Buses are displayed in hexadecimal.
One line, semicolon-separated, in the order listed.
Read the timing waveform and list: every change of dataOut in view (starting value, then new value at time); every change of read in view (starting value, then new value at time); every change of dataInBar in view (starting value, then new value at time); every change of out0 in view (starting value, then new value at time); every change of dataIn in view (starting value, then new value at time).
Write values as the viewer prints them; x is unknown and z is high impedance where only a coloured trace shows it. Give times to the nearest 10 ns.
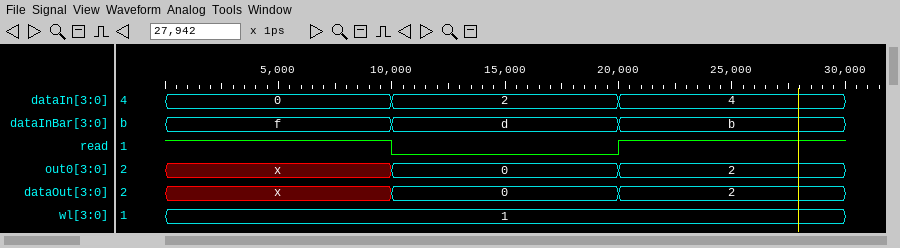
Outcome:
x, 0 at 10 ns, 2 at 20 ns; 1, 0 at 10 ns, 1 at 20 ns; f, d at 10 ns, b at 20 ns; x, 0 at 10 ns, 2 at 20 ns; 0, 2 at 10 ns, 4 at 20 ns
